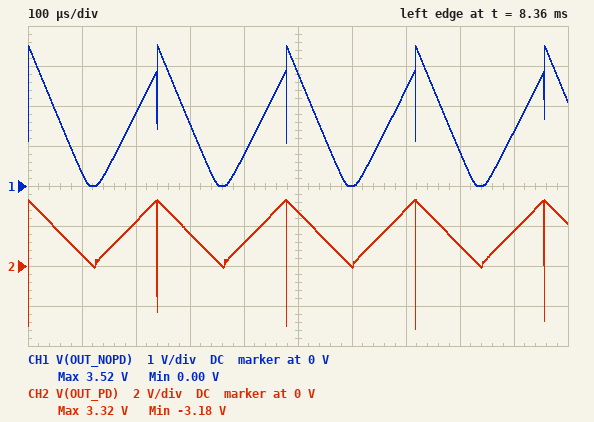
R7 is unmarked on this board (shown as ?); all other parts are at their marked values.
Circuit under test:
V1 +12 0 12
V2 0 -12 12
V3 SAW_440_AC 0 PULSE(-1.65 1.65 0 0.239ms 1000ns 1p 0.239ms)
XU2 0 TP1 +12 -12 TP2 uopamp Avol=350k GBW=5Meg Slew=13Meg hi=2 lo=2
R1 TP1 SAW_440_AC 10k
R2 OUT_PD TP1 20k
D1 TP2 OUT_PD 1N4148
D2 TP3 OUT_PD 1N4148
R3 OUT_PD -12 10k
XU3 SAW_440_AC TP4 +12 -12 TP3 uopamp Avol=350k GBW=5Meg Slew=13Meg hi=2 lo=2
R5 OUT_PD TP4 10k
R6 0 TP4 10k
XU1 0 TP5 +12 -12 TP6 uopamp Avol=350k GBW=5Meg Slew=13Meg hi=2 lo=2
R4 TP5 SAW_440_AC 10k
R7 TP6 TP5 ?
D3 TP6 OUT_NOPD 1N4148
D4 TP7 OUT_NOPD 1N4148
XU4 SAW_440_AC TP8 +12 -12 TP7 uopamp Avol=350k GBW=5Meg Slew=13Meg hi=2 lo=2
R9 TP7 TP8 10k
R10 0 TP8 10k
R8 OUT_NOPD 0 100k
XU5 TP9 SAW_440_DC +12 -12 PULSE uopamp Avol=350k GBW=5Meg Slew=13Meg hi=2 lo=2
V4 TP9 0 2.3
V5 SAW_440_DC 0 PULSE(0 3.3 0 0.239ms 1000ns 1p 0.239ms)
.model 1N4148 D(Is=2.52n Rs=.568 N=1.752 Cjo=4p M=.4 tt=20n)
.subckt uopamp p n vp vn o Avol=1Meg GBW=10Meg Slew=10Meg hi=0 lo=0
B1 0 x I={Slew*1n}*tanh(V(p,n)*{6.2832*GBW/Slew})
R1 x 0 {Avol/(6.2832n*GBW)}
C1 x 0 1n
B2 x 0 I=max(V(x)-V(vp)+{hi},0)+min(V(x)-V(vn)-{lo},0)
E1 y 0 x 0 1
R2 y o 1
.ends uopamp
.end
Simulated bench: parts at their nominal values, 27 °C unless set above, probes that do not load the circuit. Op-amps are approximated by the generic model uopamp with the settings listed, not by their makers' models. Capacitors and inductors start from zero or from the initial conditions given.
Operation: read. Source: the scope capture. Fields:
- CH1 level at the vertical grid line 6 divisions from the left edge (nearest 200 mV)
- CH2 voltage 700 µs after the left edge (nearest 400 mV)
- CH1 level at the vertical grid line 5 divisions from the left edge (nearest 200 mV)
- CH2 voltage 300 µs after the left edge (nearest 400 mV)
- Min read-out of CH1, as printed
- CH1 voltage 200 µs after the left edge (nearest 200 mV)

0 V
2.8 V
2.8 V
1.6 V
0.00 V
1.8 V
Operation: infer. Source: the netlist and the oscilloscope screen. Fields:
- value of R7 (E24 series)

24 kΩ
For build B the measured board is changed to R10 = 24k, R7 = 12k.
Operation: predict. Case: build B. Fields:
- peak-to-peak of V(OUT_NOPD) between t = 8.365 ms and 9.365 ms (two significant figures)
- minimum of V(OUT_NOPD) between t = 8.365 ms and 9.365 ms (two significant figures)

1.9 V
1.1 mV
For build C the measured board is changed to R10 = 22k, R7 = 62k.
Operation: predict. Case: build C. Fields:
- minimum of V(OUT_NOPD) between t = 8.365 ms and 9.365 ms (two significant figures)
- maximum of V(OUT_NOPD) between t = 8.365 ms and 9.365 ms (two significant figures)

-25 mV
9.5 V
